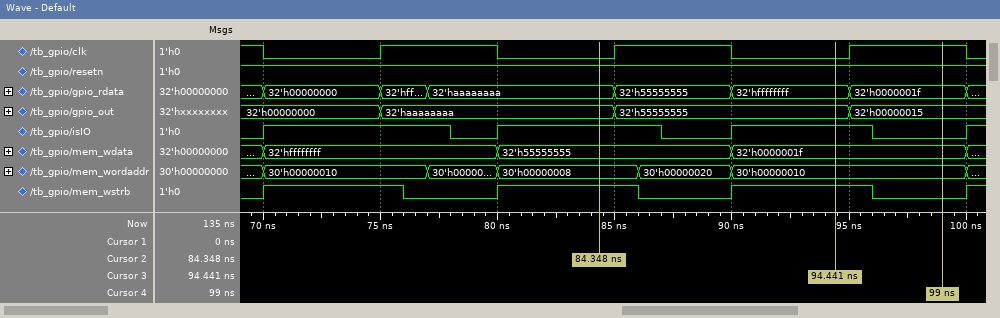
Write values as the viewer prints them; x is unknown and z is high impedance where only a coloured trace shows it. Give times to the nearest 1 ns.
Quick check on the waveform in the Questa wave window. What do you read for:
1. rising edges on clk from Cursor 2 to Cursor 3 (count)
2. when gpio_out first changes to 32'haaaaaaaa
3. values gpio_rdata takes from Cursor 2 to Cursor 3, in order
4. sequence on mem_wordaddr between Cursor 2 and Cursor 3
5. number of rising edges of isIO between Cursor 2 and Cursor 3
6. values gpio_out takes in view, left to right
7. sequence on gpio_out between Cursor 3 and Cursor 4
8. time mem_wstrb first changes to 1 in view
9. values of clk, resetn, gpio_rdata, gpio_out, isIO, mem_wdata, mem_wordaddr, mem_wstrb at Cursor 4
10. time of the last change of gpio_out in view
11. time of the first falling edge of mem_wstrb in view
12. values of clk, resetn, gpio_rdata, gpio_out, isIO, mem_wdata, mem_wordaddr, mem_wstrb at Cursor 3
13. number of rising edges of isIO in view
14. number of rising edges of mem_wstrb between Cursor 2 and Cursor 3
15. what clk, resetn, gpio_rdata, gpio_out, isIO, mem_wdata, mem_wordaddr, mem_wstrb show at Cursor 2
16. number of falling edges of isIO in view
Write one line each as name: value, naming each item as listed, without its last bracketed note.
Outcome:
rising edges on clk from Cursor 2 to Cursor 3: 1
when gpio_out first changes to 32'haaaaaaaa: 75 ns
values gpio_rdata takes from Cursor 2 to Cursor 3, in order: 32'haaaaaaaa, 32'h55555555, 32'hffffffff
sequence on mem_wordaddr between Cursor 2 and Cursor 3: 30'h00000008, 30'h00000020, 30'h00000010
number of rising edges of isIO between Cursor 2 and Cursor 3: 1
values gpio_out takes in view, left to right: 32'h00000000, 32'haaaaaaaa, 32'h55555555, 32'h00000015
sequence on gpio_out between Cursor 3 and Cursor 4: 32'h55555555, 32'h00000015
time mem_wstrb first changes to 1 in view: 70 ns
values of clk, resetn, gpio_rdata, gpio_out, isIO, mem_wdata, mem_wordaddr, mem_wstrb at Cursor 4: clk=1, resetn=1, gpio_rdata=32'h0000001f, gpio_out=32'h00000015, isIO=0, mem_wdata=32'h0000001f, mem_wordaddr=30'h00000010, mem_wstrb=0
time of the last change of gpio_out in view: 95 ns
time of the first falling edge of mem_wstrb in view: 76 ns
values of clk, resetn, gpio_rdata, gpio_out, isIO, mem_wdata, mem_wordaddr, mem_wstrb at Cursor 3: clk=0, resetn=1, gpio_rdata=32'hffffffff, gpio_out=32'h55555555, isIO=1, mem_wdata=32'h0000001f, mem_wordaddr=30'h00000010, mem_wstrb=1
number of rising edges of isIO in view: 4
number of rising edges of mem_wstrb between Cursor 2 and Cursor 3: 1
what clk, resetn, gpio_rdata, gpio_out, isIO, mem_wdata, mem_wordaddr, mem_wstrb show at Cursor 2: clk=0, resetn=1, gpio_rdata=32'haaaaaaaa, gpio_out=32'haaaaaaaa, isIO=1, mem_wdata=32'h55555555, mem_wordaddr=30'h00000008, mem_wstrb=1
number of falling edges of isIO in view: 3
